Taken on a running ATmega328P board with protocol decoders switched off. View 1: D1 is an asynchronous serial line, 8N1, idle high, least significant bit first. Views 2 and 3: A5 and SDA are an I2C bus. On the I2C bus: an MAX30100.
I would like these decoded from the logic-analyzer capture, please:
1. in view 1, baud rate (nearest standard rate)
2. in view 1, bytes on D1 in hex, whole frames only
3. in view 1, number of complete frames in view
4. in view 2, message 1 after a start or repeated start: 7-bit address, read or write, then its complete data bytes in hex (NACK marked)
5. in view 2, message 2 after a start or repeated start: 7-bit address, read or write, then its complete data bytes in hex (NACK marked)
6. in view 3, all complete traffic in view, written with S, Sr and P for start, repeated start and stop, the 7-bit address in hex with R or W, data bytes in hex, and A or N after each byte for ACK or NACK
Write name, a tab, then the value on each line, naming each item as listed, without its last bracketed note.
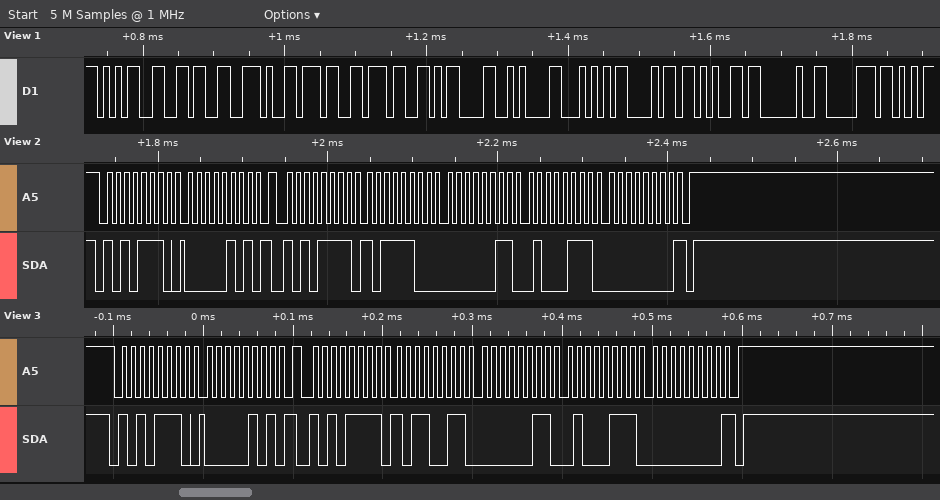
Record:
in view 1, baud rate	115200 baud
in view 1, bytes on D1 in hex, whole frames only	35 36 2E 37 37 0D 0A 54 68 65 20 70
in view 1, number of complete frames in view	12
in view 2, message 1 after a start or repeated start: 7-bit address, read or write, then its complete data bytes in hex	0x57 write: 05
in view 2, message 2 after a start or repeated start: 7-bit address, read or write, then its complete data bytes in hex	0x57 read: BC 03 47 00 NACK
in view 3, all complete traffic in view, written with S, Sr and P for start, repeated start and stop, the 7-bit address in hex with R or W, data bytes in hex, and A or N after each byte for ACK or NACK	S 57W A 05 A Sr 57R A B3 A 03 A 47 A 00 N P
